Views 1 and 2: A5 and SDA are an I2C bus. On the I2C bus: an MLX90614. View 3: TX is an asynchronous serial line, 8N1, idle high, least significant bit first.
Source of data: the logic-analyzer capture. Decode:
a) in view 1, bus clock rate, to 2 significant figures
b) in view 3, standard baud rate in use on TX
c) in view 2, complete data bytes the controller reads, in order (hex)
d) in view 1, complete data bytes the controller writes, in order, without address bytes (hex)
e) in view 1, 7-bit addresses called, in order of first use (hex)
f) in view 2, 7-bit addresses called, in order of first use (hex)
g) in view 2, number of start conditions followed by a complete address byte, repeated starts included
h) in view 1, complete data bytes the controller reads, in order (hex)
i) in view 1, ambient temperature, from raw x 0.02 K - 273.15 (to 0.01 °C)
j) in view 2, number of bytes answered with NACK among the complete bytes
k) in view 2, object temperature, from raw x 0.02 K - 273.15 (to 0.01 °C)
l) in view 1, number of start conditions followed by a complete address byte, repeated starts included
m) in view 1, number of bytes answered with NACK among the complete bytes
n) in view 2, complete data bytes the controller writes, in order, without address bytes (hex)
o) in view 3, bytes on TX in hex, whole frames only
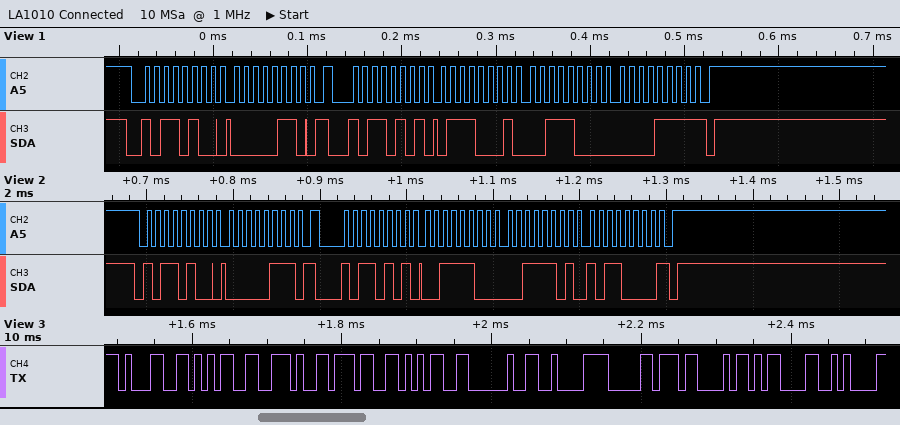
100 kHz
115200 baud
3C 3D B0
06
0x5A
0x5A
2
71 38 0F
15.83 °C
1
40.37 °C
2
1
07
0x31 0x35 0x2E 0x37 0x35 0x20 0xC2 0xB0 0x43 0x0D 0x0A
